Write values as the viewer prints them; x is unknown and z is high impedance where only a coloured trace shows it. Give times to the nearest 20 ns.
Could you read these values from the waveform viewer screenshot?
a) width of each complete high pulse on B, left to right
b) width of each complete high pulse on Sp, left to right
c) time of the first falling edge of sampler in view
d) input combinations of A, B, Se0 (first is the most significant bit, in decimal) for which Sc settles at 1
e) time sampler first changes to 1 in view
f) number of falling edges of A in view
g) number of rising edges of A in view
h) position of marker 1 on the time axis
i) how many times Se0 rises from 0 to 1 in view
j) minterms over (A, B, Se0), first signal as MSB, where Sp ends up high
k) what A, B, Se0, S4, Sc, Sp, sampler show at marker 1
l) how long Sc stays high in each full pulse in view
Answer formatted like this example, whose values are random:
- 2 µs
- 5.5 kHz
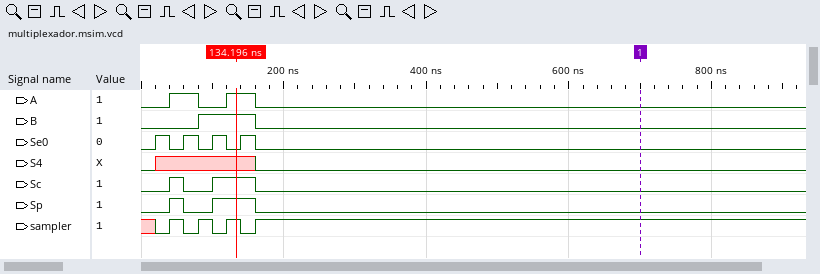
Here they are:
- 80 ns
- 20 ns, 60 ns
- 60 ns
- 3, 4, 6, 7
- 40 ns
- 2
- 2
- 700 ns
- 4
- 3, 4, 6, 7
- A=0, B=0, Se0=0, S4=0, Sc=0, Sp=0, sampler=1
- 20 ns, 60 ns
